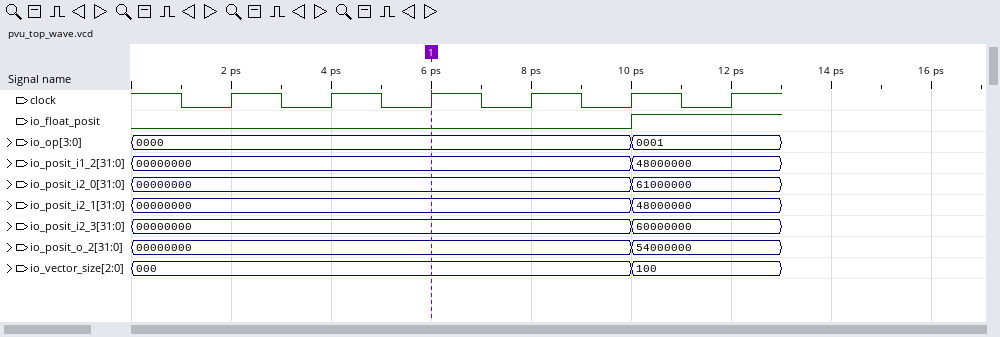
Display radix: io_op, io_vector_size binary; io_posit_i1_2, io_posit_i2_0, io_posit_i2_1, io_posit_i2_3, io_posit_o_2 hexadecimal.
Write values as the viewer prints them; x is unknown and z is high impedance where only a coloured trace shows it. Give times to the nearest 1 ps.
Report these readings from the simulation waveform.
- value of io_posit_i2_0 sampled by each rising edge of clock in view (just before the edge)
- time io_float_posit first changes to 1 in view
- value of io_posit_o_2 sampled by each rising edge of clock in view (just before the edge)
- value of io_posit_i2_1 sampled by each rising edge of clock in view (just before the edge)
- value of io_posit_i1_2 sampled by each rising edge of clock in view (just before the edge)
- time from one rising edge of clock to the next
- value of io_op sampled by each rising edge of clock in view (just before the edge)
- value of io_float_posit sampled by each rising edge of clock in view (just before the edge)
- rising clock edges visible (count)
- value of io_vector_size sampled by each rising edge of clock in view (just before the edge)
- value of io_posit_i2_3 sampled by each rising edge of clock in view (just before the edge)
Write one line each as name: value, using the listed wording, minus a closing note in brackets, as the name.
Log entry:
value of io_posit_i2_0 sampled by each rising edge of clock in view: 00000000, 00000000, 00000000, 00000000, 00000000, 61000000
time io_float_posit first changes to 1 in view: 10 ps
value of io_posit_o_2 sampled by each rising edge of clock in view: 00000000, 00000000, 00000000, 00000000, 00000000, 54000000
value of io_posit_i2_1 sampled by each rising edge of clock in view: 00000000, 00000000, 00000000, 00000000, 00000000, 48000000
value of io_posit_i1_2 sampled by each rising edge of clock in view: 00000000, 00000000, 00000000, 00000000, 00000000, 48000000
time from one rising edge of clock to the next: 2 ps
value of io_op sampled by each rising edge of clock in view: 0000, 0000, 0000, 0000, 0000, 0001
value of io_float_posit sampled by each rising edge of clock in view: 0 0 0 0 0 1
rising clock edges visible: 6
value of io_vector_size sampled by each rising edge of clock in view: 000, 000, 000, 000, 000, 100
value of io_posit_i2_3 sampled by each rising edge of clock in view: 00000000, 00000000, 00000000, 00000000, 00000000, 60000000
